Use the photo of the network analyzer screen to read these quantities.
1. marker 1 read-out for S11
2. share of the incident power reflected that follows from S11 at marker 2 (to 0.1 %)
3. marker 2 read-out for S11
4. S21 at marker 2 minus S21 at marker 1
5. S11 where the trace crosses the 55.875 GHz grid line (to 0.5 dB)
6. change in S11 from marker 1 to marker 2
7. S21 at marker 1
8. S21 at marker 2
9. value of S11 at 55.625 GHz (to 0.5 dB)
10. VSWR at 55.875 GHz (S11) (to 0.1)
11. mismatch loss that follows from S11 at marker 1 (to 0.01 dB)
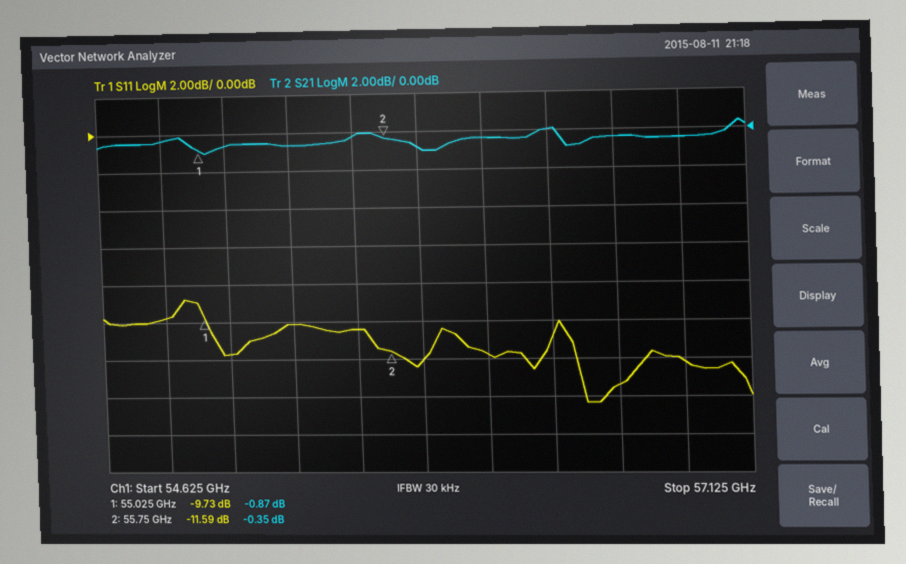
-9.73 dB
6.9 %
-11.59 dB
0.52 dB
-12.0 dB
-1.86 dB
-0.87 dB
-0.35 dB
-10.5 dB
1.7
0.49 dB
